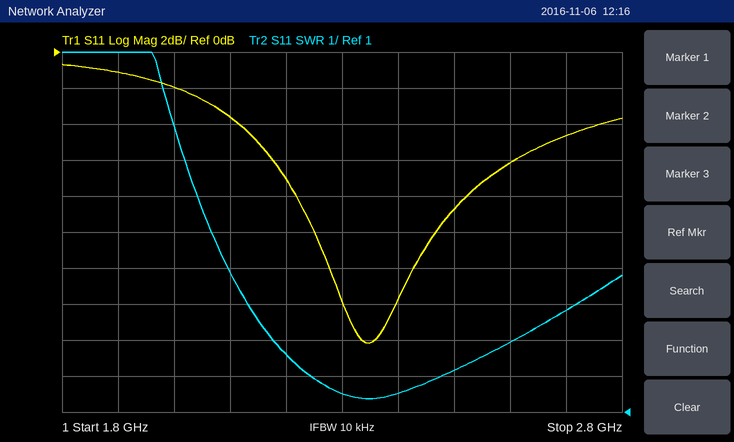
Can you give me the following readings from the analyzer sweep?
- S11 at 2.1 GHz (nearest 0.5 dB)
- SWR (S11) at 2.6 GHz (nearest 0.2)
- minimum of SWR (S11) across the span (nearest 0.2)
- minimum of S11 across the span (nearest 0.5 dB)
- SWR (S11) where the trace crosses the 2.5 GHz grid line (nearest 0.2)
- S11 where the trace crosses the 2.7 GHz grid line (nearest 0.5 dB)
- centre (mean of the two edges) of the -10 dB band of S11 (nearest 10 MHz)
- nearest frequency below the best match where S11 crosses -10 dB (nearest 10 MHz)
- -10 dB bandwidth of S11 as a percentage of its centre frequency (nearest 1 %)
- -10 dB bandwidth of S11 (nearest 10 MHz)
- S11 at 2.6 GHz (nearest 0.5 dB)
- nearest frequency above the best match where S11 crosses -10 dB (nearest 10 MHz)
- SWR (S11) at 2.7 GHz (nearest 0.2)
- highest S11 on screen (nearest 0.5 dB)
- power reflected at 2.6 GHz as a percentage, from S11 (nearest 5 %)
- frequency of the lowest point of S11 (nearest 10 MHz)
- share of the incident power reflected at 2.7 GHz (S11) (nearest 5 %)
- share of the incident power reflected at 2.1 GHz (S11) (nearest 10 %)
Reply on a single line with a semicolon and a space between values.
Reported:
-3.5 dB; 3.0; 1.4; -16.0 dB; 2.2; -4.5 dB; 2.36 GHz; 2.25 GHz; 9 %; 220 MHz; -6.0 dB; 2.47 GHz; 3.8; -0.5 dB; 25 %; 2.35 GHz; 35 %; 40 %
